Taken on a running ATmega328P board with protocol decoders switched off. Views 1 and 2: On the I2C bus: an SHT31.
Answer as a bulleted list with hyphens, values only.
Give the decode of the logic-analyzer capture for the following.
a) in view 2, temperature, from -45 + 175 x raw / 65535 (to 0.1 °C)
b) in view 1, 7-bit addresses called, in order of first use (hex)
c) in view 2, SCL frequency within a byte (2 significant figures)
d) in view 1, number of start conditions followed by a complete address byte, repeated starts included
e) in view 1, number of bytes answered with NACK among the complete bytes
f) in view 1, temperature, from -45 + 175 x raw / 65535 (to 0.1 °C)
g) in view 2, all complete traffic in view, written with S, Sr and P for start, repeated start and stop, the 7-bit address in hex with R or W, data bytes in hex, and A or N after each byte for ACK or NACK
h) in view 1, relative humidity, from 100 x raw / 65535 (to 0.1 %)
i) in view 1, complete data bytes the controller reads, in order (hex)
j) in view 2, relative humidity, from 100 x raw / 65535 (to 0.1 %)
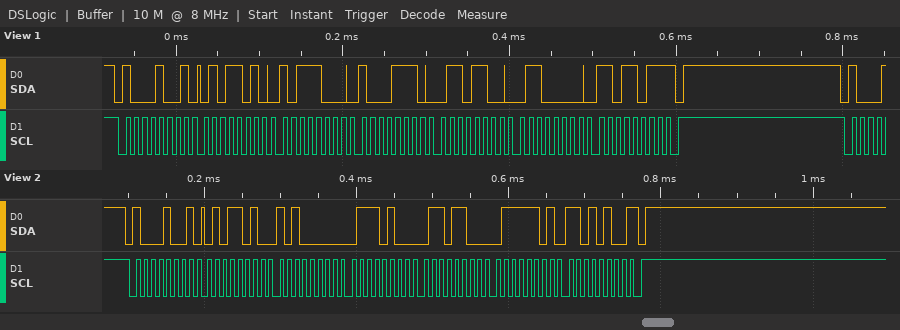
- 17.0 °C
- 0x44
- 100 kHz
- 1
- 1
- 17.0 °C
- S 44R A 5A A A0 A 74 A 6C A 7D A D4 N P
- 42.3 %
- 5A B8 8E 6C 60 DB
- 42.4 %
